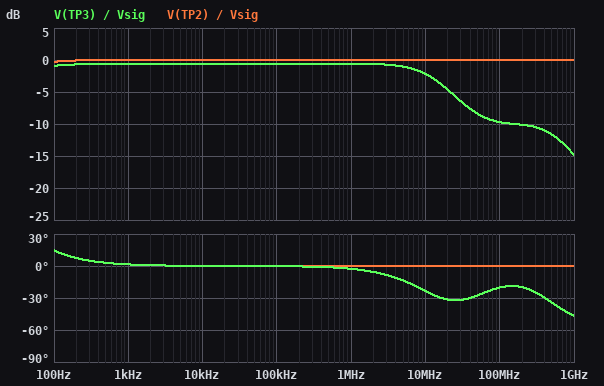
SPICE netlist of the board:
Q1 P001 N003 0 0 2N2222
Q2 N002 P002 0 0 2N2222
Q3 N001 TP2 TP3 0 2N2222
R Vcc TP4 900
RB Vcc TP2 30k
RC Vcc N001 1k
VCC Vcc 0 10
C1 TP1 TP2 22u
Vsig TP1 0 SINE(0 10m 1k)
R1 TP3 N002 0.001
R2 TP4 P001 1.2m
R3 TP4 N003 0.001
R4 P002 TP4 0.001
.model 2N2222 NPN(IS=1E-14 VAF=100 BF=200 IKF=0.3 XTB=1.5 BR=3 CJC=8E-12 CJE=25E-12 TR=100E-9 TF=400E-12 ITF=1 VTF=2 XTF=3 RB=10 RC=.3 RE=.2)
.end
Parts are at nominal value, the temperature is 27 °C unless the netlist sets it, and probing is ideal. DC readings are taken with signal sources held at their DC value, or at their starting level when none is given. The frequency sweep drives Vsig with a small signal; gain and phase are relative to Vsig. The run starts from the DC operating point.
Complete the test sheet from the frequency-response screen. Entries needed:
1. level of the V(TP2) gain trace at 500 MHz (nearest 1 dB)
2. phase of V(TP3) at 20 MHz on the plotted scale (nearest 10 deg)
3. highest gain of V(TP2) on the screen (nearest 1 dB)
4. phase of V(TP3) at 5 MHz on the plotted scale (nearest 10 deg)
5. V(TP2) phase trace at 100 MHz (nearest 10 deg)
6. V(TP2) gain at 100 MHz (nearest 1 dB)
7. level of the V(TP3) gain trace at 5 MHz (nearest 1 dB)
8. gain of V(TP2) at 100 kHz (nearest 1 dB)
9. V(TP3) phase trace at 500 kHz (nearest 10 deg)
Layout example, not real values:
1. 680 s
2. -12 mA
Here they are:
1. 0 dB
2. -30 deg
3. 0 dB
4. -10 deg
5. 0 deg
6. 0 dB
7. -1 dB
8. 0 dB
9. 0 deg
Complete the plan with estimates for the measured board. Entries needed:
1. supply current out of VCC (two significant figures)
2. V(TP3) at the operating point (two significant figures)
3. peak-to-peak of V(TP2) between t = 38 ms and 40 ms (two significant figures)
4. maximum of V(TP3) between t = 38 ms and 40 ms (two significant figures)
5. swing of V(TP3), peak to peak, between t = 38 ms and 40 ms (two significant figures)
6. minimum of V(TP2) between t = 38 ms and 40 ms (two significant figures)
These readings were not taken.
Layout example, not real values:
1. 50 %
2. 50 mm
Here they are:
1. 20 mA
2. 160 mV
3. 20 mV
4. 170 mV
5. 19 mV
6. 870 mV
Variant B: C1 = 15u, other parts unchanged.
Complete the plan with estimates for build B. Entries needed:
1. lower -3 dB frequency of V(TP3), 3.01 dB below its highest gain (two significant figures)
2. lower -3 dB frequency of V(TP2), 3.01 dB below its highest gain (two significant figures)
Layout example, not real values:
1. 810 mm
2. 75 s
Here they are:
1. 39 Hz
2. 38 Hz
